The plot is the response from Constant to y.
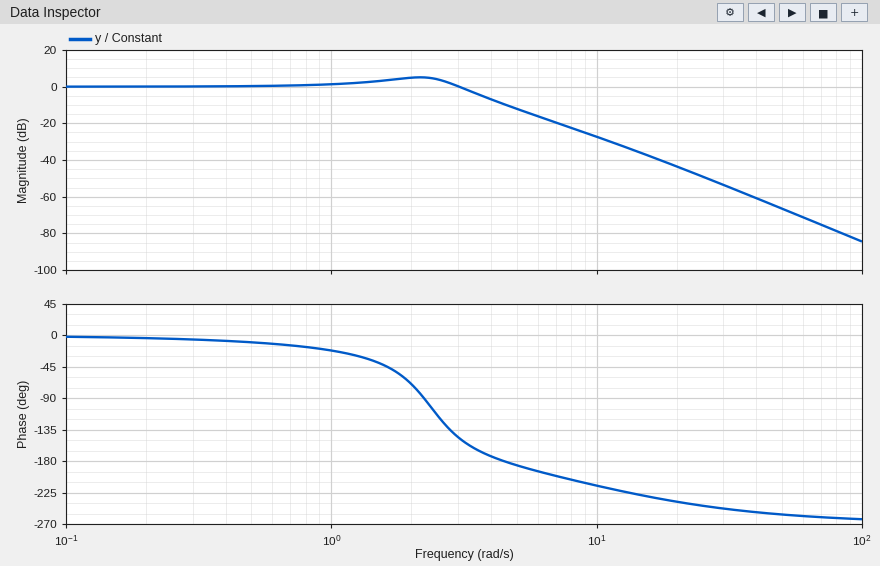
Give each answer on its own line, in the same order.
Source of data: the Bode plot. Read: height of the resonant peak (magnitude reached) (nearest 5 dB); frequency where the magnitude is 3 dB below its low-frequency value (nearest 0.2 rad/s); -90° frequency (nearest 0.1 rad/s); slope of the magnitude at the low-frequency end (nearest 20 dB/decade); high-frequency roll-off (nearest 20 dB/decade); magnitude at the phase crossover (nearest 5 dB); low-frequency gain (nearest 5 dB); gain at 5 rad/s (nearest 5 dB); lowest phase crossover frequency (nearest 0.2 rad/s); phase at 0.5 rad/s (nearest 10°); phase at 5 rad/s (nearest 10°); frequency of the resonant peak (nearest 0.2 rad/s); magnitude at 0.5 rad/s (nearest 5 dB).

5 dB
3.4 rad/s
2.2 rad/s
0 dB/decade
-60 dB/decade
-10 dB
0 dB
-10 dB
4.4 rad/s
-10°
-190°
2.2 rad/s
0 dB
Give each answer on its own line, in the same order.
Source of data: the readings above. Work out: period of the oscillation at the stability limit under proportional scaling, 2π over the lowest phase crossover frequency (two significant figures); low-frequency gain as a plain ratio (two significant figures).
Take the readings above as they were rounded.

1.4 s
1.0
